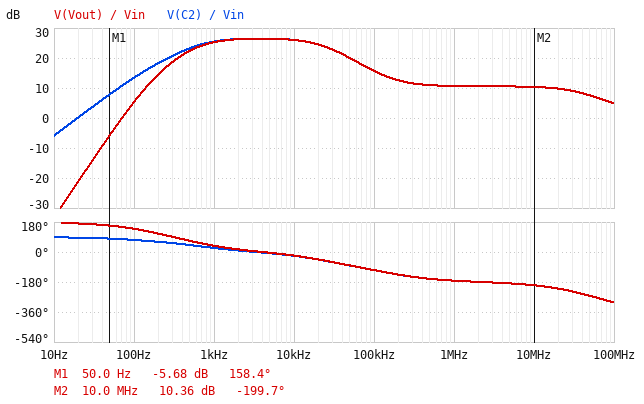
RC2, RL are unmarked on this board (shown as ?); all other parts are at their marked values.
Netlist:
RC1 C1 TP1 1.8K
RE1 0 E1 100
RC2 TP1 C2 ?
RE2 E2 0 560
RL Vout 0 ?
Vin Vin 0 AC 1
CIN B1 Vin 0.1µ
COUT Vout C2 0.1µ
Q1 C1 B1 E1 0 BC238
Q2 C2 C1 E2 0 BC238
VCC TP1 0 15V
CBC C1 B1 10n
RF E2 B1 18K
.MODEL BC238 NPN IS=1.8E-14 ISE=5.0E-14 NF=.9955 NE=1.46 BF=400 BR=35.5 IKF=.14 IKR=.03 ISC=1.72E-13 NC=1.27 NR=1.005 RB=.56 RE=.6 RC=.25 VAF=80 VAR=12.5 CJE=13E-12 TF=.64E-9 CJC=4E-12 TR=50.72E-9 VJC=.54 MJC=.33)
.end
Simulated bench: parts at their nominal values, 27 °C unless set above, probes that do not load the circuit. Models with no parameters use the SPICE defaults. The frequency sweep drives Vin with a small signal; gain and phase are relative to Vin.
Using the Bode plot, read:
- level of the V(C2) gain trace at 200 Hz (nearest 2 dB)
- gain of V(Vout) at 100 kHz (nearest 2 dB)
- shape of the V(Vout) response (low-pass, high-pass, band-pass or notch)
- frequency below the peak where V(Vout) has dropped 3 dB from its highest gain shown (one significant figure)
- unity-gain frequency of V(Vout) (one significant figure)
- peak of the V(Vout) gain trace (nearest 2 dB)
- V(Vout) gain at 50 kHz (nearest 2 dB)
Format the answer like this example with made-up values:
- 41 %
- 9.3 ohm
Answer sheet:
- 18 dB
- 16 dB
- band-pass
- 600 Hz
- 70 Hz
- 26 dB
- 20 dB
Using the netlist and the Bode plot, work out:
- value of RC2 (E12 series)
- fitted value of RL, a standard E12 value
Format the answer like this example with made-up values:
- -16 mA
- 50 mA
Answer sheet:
- 2.7 kΩ
- 6.8 kΩ
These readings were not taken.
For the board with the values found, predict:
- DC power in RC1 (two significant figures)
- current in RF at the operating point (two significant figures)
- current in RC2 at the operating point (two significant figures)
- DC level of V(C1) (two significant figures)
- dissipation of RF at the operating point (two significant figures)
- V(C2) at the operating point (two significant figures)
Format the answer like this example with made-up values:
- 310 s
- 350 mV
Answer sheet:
- 87 mW
- 23 µA
- 3.2 mA
- 2.5 V
- 9.8 µW
- 6.2 V
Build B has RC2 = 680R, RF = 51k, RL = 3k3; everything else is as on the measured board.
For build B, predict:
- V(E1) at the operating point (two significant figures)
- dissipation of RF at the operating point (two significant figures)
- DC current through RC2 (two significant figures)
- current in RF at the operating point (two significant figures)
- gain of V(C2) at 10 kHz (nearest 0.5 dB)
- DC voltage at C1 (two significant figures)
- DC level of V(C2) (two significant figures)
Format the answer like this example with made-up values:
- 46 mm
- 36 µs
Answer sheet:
- 660 mV
- 24 µW
- 4.4 mA
- 22 µA
- 15.0 dB
- 3.1 V
- 12 V
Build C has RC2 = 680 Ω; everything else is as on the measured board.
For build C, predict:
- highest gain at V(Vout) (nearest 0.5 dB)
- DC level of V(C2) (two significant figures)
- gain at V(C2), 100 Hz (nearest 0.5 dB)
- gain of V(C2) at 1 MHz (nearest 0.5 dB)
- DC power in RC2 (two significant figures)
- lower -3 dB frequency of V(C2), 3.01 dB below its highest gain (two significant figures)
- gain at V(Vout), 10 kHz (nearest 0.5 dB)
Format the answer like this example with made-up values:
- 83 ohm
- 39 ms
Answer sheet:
- 16.5 dB
- 13 V
- 2.0 dB
- 1.0 dB
- 7.2 mW
- 550 Hz
- 16.0 dB
